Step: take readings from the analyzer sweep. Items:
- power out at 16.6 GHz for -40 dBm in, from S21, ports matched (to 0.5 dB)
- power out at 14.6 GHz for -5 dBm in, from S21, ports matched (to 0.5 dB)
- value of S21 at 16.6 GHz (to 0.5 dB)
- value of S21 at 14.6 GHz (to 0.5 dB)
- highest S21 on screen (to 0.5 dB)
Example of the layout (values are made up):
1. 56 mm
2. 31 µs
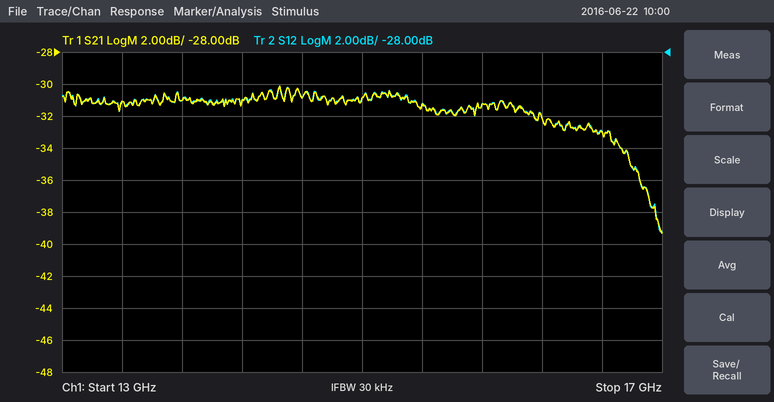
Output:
1. -73.0 dBm
2. -36.0 dBm
3. -33.0 dB
4. -31.0 dB
5. -30.0 dB
